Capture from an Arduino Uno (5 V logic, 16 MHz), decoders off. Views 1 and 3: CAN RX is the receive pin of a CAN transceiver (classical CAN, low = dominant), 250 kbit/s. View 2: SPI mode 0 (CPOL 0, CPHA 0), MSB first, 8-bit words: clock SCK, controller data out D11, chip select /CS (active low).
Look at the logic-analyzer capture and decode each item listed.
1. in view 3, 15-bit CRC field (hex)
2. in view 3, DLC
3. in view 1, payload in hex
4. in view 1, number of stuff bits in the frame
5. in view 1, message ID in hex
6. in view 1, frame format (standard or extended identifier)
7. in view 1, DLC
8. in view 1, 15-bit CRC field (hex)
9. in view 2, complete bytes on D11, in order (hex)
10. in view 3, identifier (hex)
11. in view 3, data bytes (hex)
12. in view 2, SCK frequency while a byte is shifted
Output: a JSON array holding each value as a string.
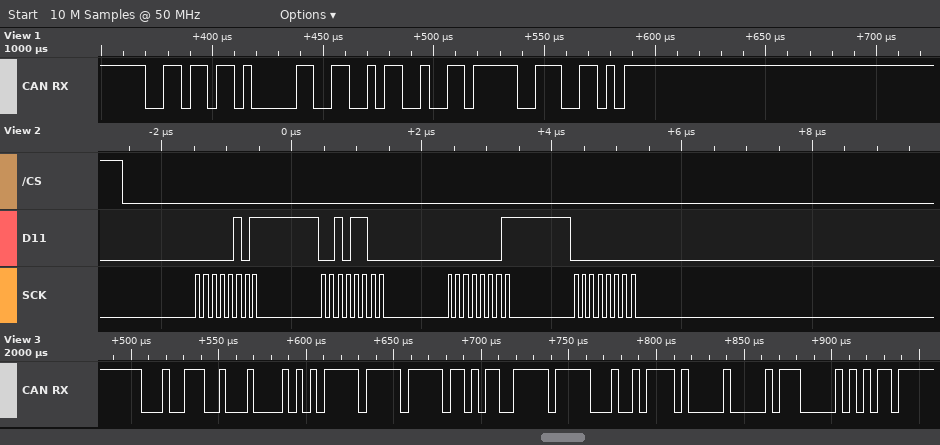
["0x3815", "8", "65 93", "2", "0x36D", "standard", "2", "0x3EE6", "0x05 0x2C 0x01 0x00", "0x139", "55 FF FF 59 FF 92 F4 00", "8 MHz"]
